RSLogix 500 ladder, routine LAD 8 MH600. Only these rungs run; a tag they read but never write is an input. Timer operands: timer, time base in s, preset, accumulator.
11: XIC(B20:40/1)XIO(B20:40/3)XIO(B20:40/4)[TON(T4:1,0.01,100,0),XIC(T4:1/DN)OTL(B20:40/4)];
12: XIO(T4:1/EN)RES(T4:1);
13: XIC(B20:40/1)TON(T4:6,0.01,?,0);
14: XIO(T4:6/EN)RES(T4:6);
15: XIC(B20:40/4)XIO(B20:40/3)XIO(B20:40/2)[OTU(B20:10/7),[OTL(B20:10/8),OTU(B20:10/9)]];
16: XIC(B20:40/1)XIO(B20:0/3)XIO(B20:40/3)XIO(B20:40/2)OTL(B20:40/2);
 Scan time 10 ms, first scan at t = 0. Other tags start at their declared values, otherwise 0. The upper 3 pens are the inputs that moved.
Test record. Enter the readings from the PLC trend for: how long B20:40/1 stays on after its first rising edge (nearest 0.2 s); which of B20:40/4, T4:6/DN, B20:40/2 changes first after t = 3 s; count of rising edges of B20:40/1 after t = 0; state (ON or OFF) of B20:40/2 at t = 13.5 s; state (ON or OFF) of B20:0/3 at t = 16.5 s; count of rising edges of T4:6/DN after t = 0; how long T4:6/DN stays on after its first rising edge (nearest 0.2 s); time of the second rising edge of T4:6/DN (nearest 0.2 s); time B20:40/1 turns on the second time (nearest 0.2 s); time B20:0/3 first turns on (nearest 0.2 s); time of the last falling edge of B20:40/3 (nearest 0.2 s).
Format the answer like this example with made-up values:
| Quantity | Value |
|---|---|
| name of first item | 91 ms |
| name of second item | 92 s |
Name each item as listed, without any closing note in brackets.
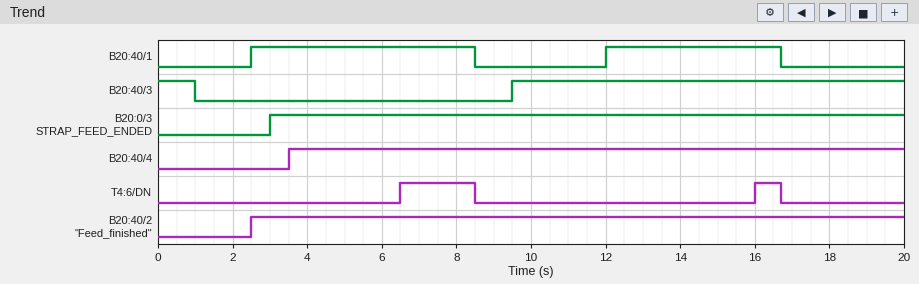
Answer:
| Quantity | Value |
|---|---|
| how long B20:40/1 stays on after its first rising edge | 6.0 s |
| which of B20:40/4, T4:6/DN, B20:40/2 changes first after t = 3 s | B20:40/4 |
| count of rising edges of B20:40/1 after t = 0 | 2 |
| state (ON or OFF) of B20:40/2 at t = 13.5 s | ON |
| state (ON or OFF) of B20:0/3 at t = 16.5 s | ON |
| count of rising edges of T4:6/DN after t = 0 | 2 |
| how long T4:6/DN stays on after its first rising edge | 2.0 s |
| time of the second rising edge of T4:6/DN | 16.0 s |
| time B20:40/1 turns on the second time | 12.0 s |
| time B20:0/3 first turns on | 3.0 s |
| time of the last falling edge of B20:40/3 | 1.0 s |
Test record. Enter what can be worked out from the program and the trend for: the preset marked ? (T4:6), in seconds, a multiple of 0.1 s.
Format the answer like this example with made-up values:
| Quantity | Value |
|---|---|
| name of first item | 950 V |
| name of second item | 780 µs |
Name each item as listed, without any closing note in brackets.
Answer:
| Quantity | Value |
|---|---|
| the preset marked ? (T4:6), in seconds, a multiple of 0.1 s | 4.0 s |
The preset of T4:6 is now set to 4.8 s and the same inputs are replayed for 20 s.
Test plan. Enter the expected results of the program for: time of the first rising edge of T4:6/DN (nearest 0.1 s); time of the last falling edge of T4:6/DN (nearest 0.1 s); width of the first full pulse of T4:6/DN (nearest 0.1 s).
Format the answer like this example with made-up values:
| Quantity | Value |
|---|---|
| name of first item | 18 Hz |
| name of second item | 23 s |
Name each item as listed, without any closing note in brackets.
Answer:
| Quantity | Value |
|---|---|
| time of the first rising edge of T4:6/DN | 7.3 s |
| time of the last falling edge of T4:6/DN | 8.5 s |
| width of the first full pulse of T4:6/DN | 1.2 s |
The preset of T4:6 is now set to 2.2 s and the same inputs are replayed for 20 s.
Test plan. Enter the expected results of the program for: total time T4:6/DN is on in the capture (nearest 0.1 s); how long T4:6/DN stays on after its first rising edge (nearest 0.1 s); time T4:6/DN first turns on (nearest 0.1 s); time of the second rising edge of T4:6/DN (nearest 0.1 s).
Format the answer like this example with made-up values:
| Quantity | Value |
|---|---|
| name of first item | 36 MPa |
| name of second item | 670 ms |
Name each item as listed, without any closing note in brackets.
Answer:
| Quantity | Value |
|---|---|
| total time T4:6/DN is on in the capture | 6.3 s |
| how long T4:6/DN stays on after its first rising edge | 3.8 s |
| time T4:6/DN first turns on | 4.7 s |
| time of the second rising edge of T4:6/DN | 14.2 s |
